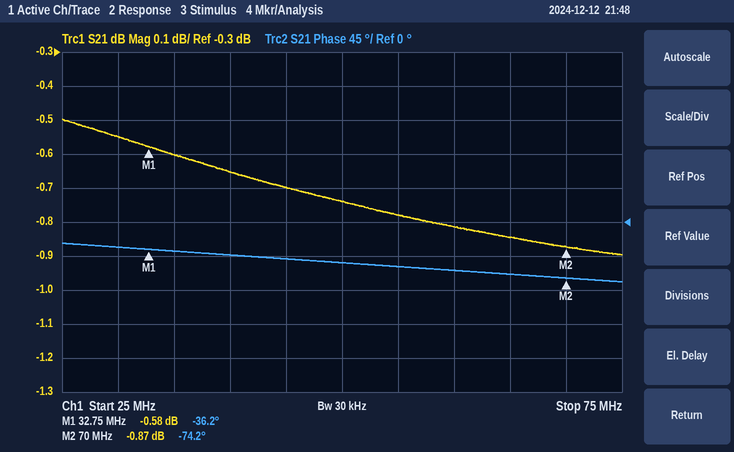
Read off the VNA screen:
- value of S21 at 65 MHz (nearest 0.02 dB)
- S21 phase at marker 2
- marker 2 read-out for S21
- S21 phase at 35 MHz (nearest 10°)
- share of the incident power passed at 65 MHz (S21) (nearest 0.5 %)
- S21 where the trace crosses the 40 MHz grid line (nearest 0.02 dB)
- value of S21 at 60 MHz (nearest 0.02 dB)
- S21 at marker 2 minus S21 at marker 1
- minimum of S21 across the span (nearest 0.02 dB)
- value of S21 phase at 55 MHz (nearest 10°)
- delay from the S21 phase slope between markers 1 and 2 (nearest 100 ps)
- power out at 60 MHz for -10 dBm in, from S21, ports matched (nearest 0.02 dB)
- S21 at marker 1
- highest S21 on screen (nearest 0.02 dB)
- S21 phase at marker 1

-0.84 dB
-74.2°
-0.87 dB
-40°
82.5 %
-0.66 dB
-0.82 dB
-0.29 dB
-0.90 dB
-60°
2.8 ns
-10.82 dBm
-0.58 dB
-0.50 dB
-36.2°
